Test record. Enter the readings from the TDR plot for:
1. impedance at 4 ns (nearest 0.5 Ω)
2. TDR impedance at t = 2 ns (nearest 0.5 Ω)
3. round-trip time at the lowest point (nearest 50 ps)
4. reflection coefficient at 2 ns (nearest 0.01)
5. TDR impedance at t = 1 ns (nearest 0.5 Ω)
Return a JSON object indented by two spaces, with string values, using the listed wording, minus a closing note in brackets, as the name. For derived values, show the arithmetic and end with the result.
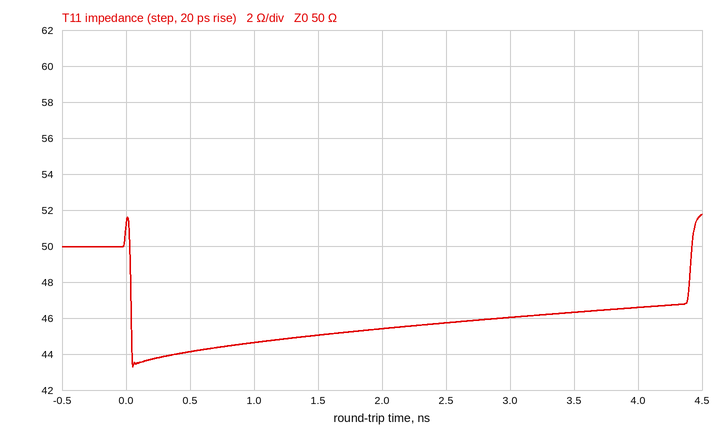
{
  "impedance at 4 ns": "46.5 Ω",
  "TDR impedance at t = 2 ns": "45.5 Ω",
  "round-trip time at the lowest point": "50 ps",
  "reflection coefficient at 2 ns": "(45.5 − 50)/(45.5 + 50) ≈ -0.05",
  "TDR impedance at t = 1 ns": "44.5 Ω"
}
